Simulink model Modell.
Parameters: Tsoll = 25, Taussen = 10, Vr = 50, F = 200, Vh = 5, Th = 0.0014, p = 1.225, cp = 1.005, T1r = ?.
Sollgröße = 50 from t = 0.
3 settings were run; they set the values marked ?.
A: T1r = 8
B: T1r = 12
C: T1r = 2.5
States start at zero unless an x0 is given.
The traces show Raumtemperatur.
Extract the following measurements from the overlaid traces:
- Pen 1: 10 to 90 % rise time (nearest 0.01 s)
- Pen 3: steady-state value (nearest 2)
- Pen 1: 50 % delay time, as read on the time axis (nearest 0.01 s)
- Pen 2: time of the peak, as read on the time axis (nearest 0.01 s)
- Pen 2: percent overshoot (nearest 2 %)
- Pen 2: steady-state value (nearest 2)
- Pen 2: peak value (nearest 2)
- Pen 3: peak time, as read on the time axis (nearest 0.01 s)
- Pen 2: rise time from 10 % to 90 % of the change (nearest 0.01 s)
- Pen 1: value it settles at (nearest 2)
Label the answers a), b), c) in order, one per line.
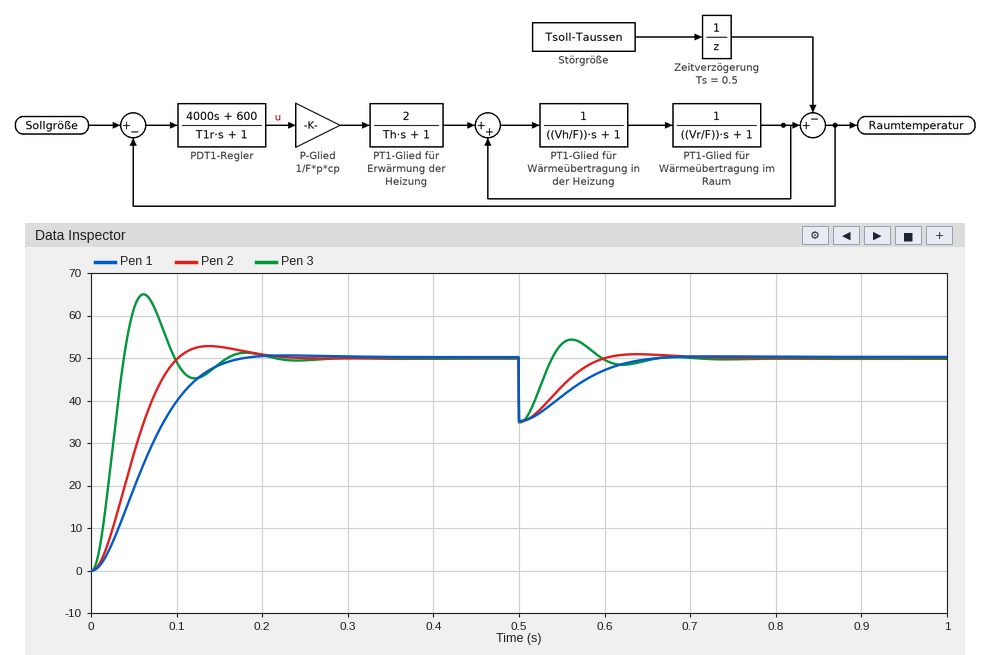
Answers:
a) 0.10 s
b) 50
c) 0.06 s
d) 0.14 s
e) 6 %
f) 50
g) 52
h) 0.06 s
i) 0.07 s
j) 50
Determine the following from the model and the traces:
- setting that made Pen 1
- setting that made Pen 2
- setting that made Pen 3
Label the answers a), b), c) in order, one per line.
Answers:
a) B
b) A
c) C
